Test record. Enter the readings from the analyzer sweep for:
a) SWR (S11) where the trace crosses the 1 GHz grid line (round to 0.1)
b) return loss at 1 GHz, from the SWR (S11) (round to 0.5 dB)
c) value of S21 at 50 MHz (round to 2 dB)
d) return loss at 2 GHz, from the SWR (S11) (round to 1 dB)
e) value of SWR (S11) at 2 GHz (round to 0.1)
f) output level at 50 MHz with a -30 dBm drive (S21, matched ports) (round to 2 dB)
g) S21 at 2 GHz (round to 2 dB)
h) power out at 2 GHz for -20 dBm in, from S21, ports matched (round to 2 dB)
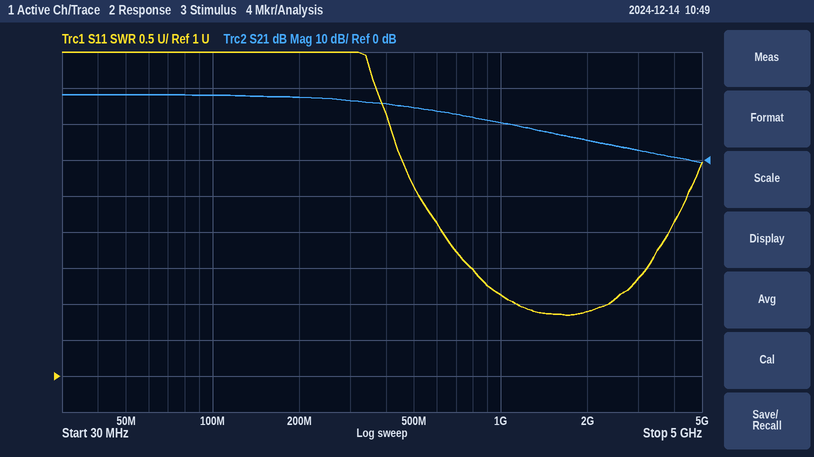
2.1
9.0 dB
18 dB
10 dB
1.9
-12 dBm
6 dB
-14 dBm
